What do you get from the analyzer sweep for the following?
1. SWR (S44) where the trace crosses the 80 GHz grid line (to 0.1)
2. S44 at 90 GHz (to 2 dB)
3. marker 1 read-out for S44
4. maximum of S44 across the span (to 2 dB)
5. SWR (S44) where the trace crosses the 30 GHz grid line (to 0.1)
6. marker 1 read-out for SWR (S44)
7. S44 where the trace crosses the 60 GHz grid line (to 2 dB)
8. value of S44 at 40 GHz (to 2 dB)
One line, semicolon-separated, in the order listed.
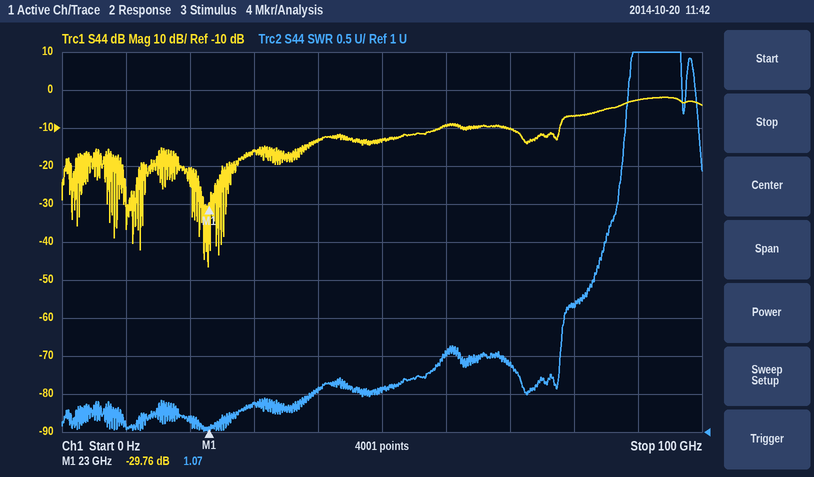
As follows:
2.7; -2 dB; -29.76 dB; -2 dB; 1.4; 1.07; -10 dB; -14 dB
